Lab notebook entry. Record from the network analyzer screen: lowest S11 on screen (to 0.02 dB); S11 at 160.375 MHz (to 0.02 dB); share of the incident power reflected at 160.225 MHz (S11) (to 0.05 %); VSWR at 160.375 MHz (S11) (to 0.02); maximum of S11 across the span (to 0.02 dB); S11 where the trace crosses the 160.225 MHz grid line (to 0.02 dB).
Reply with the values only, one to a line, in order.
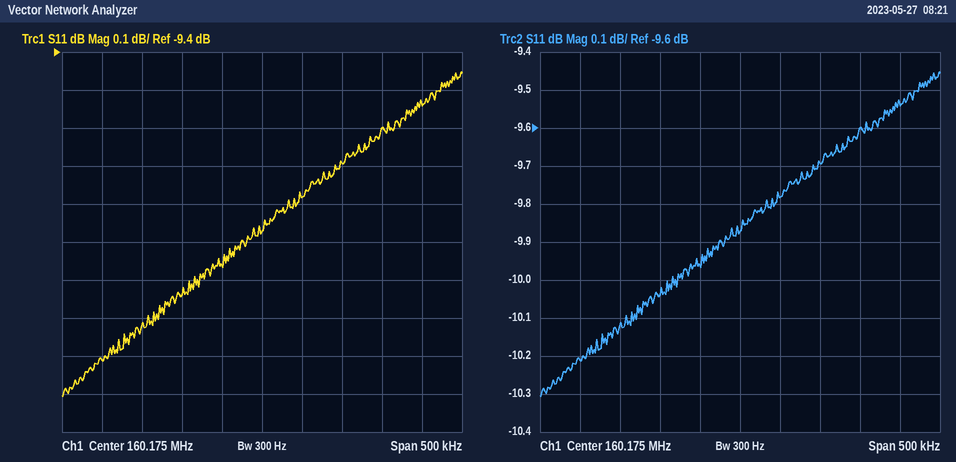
-10.30 dB
-9.54 dB
10.50 %
2.00
-9.46 dB
-9.78 dB
